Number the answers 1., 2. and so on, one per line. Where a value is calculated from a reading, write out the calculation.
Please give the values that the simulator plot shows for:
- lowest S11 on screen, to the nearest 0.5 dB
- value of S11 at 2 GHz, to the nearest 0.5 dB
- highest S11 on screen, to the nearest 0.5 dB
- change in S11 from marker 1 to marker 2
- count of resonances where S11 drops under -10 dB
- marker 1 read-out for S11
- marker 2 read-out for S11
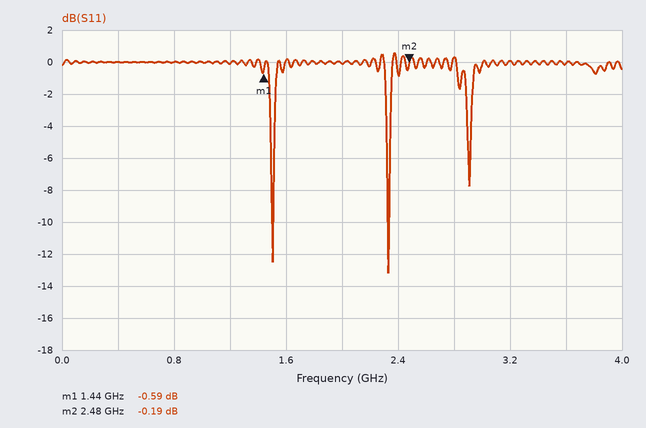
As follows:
1. -13.0 dB
2. 0.0 dB
3. 0.5 dB
4. -0.19 − (-0.59) = 0.40 dB
5. 2
6. -0.59 dB
7. -0.19 dB
